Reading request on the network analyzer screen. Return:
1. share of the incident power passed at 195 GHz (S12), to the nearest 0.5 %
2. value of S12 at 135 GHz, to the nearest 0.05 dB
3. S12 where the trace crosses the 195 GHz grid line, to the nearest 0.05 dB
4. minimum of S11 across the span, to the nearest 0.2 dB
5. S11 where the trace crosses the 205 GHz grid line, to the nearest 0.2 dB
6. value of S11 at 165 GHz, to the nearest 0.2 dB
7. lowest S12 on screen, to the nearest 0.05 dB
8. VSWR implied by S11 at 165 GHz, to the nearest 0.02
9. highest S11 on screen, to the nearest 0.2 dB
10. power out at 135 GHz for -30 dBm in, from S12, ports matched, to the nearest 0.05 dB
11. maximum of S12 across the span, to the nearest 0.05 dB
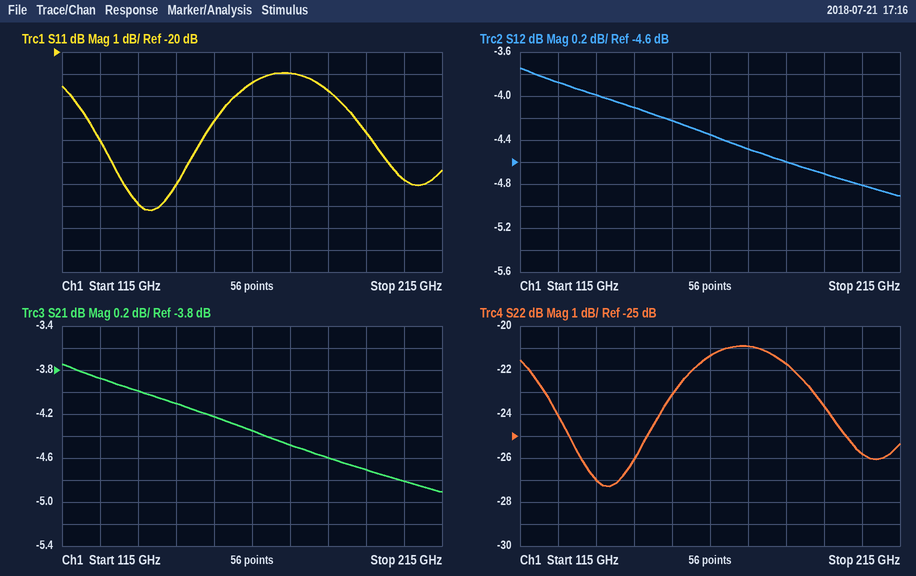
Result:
34.0 %
-4.00 dB
-4.70 dB
-27.2 dB
-25.8 dB
-21.4 dB
-4.90 dB
1.18
-21.0 dB
-34.00 dBm
-3.75 dB
